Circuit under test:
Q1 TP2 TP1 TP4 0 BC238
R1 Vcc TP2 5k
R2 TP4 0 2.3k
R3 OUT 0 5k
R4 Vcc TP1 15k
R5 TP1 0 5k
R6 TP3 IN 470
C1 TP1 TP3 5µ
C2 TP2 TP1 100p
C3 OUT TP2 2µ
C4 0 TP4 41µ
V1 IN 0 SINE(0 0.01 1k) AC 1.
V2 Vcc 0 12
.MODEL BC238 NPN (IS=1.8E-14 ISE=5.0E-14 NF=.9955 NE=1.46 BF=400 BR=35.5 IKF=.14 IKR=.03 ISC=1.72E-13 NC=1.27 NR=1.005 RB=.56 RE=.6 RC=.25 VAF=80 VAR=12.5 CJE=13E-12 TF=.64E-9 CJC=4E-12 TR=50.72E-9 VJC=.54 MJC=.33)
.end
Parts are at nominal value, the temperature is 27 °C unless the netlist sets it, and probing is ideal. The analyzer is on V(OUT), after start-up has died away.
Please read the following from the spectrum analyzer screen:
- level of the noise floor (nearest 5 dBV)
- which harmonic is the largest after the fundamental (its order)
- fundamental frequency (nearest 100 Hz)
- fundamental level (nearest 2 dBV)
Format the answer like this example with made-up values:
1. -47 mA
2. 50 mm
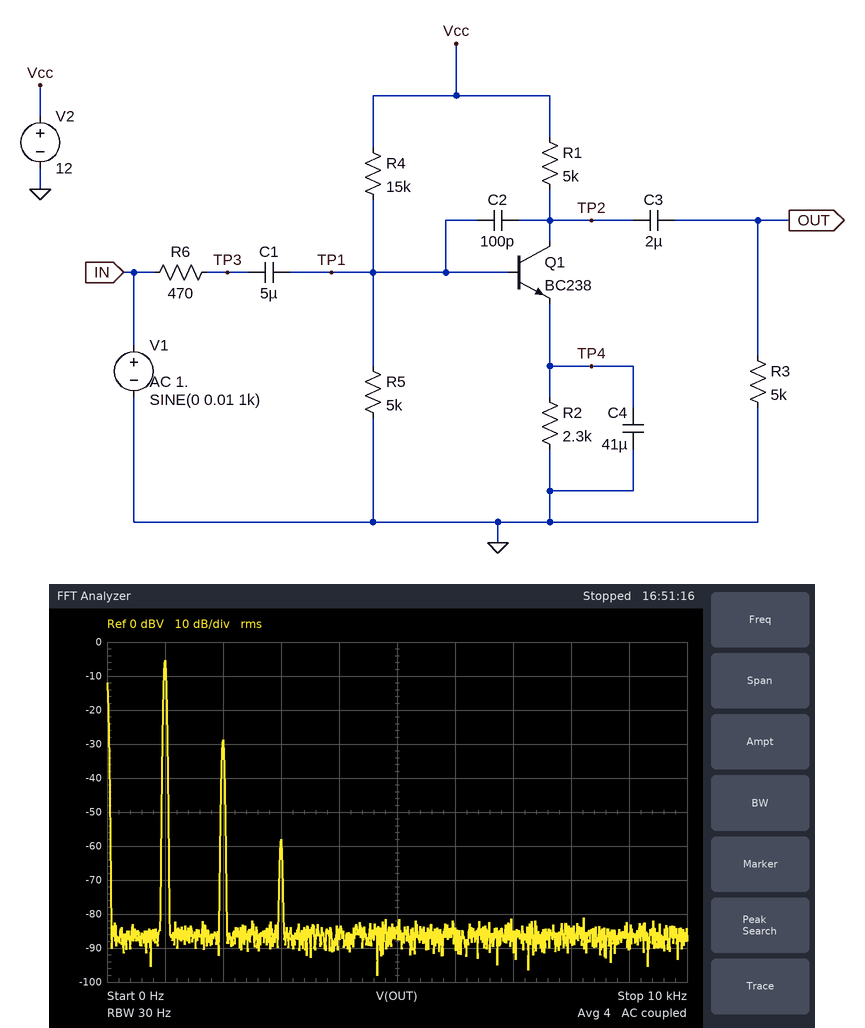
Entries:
1. -85 dBV
2. 2
3. 1.0 kHz
4. -6 dBV
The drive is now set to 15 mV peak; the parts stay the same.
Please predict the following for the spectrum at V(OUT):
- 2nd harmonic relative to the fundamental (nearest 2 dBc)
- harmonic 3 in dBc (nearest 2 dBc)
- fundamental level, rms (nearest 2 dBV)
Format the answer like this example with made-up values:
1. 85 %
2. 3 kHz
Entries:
1. -20 dBc
2. -46 dBc
3. -2 dBV
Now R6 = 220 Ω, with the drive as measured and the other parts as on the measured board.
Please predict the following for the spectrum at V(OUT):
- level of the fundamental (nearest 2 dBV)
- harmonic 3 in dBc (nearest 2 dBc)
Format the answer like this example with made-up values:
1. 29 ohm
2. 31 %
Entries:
1. -4 dBV
2. -50 dBc
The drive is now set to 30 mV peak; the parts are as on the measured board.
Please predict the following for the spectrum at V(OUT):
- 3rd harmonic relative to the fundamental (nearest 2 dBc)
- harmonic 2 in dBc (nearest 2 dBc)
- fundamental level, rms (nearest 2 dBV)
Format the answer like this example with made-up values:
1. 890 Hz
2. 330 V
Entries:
1. -34 dBc
2. -14 dBc
3. 4 dBV
